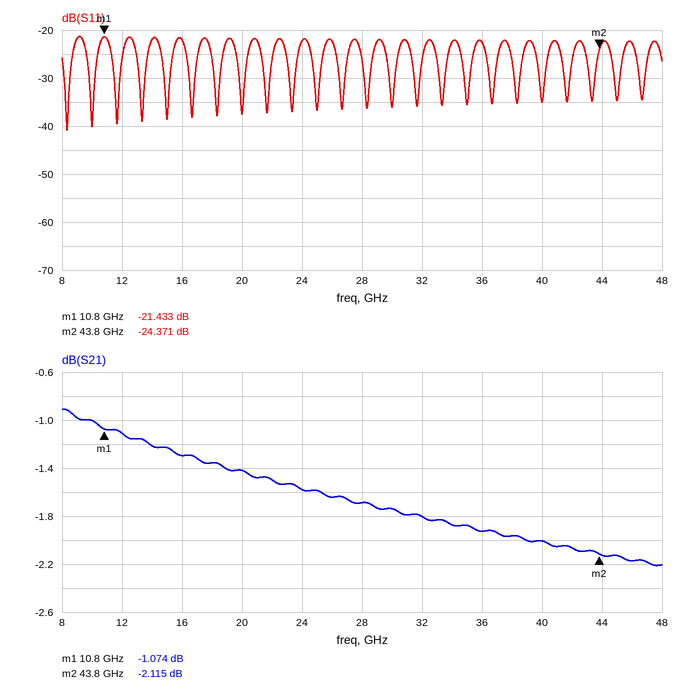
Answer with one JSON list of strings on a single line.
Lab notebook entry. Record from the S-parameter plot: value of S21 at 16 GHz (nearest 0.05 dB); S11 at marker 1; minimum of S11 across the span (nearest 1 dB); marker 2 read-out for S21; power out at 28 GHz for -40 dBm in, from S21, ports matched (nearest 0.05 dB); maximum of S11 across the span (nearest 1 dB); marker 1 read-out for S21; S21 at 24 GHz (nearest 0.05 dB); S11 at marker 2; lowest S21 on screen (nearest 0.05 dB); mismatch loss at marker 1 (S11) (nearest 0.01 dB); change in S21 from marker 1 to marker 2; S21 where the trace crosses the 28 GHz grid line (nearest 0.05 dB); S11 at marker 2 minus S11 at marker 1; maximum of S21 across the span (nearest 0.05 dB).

["-1.30 dB", "-21.433 dB", "-41 dB", "-2.115 dB", "-41.70 dBm", "-21 dB", "-1.074 dB", "-1.60 dB", "-24.371 dB", "-2.20 dB", "0.03 dB", "-1.041 dB", "-1.70 dB", "-2.938 dB", "-0.90 dB"]
